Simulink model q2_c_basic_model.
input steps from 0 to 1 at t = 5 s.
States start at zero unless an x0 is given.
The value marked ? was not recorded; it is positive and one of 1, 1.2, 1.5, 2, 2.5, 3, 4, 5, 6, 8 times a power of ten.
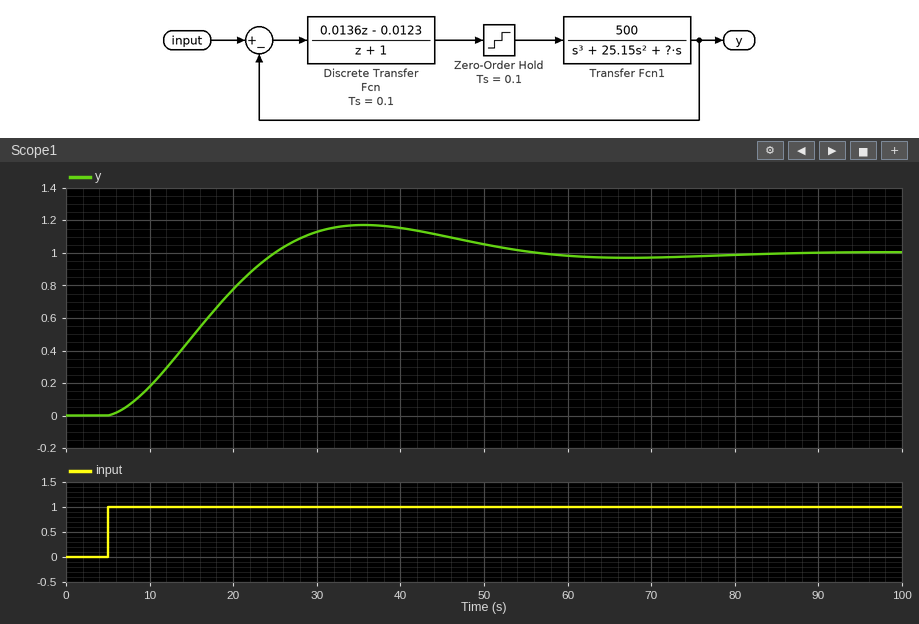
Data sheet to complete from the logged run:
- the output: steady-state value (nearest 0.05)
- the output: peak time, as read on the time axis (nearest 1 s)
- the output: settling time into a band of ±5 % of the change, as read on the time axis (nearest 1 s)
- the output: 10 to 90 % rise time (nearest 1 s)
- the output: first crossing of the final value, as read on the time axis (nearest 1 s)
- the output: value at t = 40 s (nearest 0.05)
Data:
1.00
36 s
50 s
14 s
25 s
1.15
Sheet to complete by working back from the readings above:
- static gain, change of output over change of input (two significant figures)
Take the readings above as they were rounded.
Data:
1.0
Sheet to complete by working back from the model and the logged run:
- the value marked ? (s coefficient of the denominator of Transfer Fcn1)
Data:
2.5
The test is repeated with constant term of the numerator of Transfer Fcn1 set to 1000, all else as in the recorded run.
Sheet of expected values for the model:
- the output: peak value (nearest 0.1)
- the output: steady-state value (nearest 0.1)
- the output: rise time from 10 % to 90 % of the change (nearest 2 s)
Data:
1.3
1.0
8 s
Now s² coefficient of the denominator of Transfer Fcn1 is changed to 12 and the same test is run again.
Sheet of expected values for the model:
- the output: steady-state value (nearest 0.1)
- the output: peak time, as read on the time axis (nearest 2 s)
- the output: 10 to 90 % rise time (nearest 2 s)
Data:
1.0
30 s
12 s
